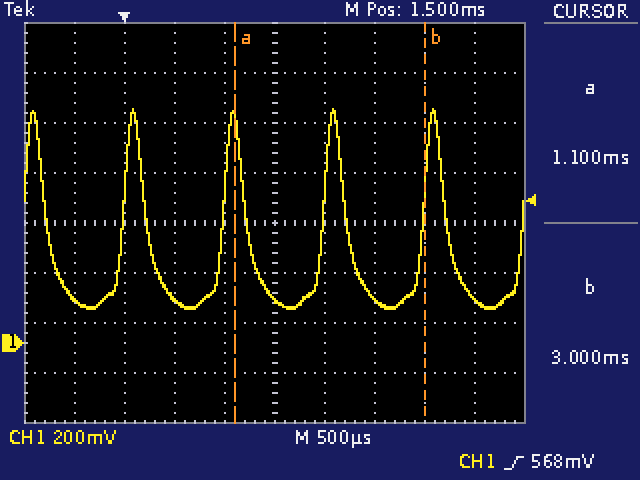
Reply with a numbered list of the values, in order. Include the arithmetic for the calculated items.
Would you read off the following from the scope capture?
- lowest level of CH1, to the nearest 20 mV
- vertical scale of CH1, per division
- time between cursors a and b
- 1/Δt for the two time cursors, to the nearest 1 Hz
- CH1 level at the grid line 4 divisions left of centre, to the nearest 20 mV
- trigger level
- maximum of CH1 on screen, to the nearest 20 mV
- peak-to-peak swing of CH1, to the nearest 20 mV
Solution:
1. 140 mV
2. 200 mV
3. 3 ms − (1.1 ms) = 1.90 ms
4. 1 / 1.90 ms ≈ 526 Hz
5. 180 mV
6. 568 mV
7. 940 mV
8. 940 mV − (140 mV) = 800 mV
